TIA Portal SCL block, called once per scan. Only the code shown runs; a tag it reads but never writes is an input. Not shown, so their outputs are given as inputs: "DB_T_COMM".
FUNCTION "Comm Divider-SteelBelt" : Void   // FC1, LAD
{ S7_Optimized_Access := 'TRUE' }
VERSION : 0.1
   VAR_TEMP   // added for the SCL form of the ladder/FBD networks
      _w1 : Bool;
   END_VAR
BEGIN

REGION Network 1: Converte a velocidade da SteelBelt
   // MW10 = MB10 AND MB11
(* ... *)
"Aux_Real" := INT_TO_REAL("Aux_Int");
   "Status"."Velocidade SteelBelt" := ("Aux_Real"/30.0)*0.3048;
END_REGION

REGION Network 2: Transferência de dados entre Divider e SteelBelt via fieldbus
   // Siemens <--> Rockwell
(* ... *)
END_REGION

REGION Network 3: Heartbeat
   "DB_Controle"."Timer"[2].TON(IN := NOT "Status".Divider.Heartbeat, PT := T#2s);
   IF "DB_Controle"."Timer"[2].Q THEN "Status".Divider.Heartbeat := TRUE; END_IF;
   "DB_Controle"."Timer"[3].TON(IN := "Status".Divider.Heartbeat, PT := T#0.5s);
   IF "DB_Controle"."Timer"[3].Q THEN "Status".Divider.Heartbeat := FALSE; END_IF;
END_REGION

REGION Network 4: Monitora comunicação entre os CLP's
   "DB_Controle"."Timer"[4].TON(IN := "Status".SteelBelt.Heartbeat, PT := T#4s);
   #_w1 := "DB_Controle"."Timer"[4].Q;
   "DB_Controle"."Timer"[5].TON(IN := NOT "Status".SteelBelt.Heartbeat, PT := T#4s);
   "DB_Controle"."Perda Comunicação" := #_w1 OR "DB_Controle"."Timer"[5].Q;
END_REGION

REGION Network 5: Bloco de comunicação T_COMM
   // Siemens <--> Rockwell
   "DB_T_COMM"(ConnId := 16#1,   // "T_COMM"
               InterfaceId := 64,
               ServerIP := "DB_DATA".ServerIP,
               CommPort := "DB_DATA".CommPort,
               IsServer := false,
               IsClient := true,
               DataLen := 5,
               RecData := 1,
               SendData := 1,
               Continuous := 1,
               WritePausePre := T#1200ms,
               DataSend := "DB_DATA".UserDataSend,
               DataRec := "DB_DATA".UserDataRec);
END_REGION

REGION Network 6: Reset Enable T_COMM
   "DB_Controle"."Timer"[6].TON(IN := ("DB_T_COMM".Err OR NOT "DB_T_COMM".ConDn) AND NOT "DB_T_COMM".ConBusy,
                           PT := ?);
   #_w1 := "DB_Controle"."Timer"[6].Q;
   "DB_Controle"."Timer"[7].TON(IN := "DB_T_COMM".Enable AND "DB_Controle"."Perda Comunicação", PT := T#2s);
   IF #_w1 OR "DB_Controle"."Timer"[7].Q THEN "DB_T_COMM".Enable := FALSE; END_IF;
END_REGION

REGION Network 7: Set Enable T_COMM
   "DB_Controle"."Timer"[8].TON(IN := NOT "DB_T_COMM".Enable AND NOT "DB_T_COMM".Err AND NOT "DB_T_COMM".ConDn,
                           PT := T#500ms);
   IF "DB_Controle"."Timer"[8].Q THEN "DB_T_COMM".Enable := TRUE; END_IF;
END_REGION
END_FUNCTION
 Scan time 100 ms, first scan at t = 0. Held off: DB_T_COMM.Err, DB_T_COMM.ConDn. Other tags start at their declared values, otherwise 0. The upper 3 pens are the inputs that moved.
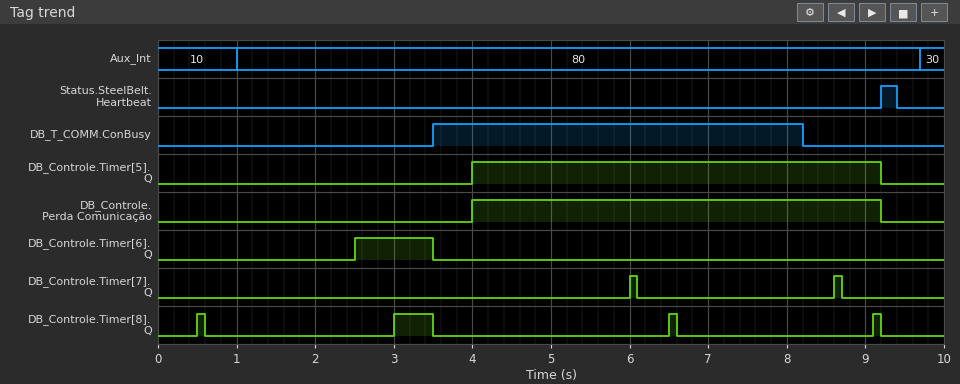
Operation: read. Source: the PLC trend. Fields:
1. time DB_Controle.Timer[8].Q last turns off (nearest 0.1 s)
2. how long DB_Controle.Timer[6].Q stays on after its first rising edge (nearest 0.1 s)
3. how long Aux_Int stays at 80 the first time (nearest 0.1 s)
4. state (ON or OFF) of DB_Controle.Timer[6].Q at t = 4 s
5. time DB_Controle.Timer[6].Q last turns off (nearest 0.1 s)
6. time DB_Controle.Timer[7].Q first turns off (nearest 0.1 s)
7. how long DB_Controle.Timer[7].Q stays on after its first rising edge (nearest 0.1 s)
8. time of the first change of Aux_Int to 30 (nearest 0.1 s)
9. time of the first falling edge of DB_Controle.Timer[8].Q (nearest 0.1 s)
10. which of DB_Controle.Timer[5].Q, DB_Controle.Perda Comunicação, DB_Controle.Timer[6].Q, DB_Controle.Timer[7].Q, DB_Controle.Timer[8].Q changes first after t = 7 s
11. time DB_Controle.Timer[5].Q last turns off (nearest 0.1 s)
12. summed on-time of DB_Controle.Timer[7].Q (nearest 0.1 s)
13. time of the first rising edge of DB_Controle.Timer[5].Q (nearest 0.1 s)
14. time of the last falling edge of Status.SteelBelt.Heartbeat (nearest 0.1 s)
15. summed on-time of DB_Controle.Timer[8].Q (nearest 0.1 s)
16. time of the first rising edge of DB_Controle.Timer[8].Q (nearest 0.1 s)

9.2 s
1.0 s
8.7 s
OFF
3.5 s
6.1 s
0.1 s
9.7 s
0.6 s
DB_Controle.Timer[7].Q
9.2 s
0.2 s
4.0 s
9.4 s
0.8 s
0.5 s
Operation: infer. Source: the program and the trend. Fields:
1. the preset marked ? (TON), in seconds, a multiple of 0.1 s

2.5 s
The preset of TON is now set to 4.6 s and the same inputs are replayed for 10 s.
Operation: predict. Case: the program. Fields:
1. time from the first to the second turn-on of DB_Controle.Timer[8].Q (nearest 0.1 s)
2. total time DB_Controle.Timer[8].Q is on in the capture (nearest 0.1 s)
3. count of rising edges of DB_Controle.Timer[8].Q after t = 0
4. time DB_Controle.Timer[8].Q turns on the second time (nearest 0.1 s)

6.0 s
0.3 s
3
6.5 s
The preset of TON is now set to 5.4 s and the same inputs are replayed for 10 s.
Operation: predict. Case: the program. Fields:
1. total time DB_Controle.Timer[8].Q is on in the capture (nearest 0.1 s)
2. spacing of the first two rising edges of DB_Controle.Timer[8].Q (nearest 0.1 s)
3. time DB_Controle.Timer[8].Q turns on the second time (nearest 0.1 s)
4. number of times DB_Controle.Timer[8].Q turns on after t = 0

0.3 s
6.0 s
6.5 s
3
